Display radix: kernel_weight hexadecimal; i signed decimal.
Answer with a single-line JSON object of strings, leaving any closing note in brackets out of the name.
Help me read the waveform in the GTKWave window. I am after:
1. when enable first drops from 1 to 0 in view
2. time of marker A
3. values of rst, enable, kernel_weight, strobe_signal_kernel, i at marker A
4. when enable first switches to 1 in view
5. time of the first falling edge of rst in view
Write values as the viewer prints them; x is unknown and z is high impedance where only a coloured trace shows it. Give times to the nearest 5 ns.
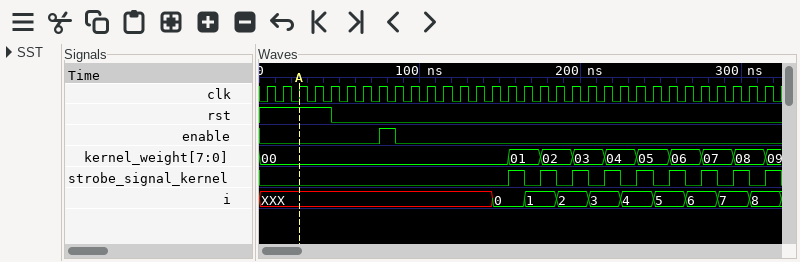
{"when enable first drops from 1 to 0 in view": "85 ns", "time of marker A": "25 ns", "values of rst, enable, kernel_weight, strobe_signal_kernel, i at marker A": "rst=1, enable=0, kernel_weight=00, strobe_signal_kernel=0, i=XXX", "when enable first switches to 1 in view": "75 ns", "time of the first falling edge of rst in view": "45 ns"}
